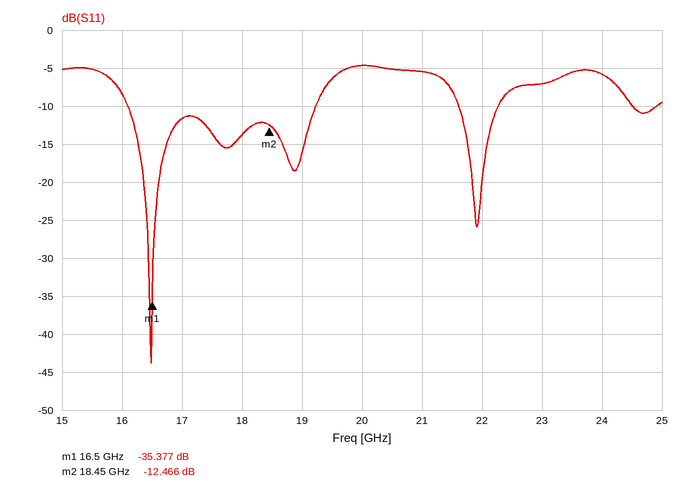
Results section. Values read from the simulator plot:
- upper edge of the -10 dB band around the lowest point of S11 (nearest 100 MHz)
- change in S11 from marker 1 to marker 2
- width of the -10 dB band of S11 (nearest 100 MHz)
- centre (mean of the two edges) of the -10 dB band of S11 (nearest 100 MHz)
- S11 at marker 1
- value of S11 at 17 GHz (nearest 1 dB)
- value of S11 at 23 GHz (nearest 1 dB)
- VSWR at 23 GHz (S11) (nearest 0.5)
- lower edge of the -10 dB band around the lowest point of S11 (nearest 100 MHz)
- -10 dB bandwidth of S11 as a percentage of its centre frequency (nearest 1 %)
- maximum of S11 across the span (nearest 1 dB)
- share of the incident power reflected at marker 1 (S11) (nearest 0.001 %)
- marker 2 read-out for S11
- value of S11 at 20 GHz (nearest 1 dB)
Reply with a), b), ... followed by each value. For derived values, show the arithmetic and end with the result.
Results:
a) 19.2 GHz
b) -12.466 − (-35.377) = 22.911 dB
c) 19.2 GHz − 16.1 GHz = 3.1 GHz
d) 17.7 GHz
e) -35.377 dB
f) -12 dB
g) -7 dB
h) |Γ| = 10^(-7/20) = 0.4467; VSWR = (1 + 0.4467)/(1 − 0.4467) ≈ 2.61, so 2.5 to the nearest 0.5
i) 16.1 GHz
j) 3.1 GHz / 17.65 GHz ≈ 18 %
k) -5 dB
l) 10^(-35.377/10) ≈ 0.029 %
m) -12.466 dB
n) -5 dB
